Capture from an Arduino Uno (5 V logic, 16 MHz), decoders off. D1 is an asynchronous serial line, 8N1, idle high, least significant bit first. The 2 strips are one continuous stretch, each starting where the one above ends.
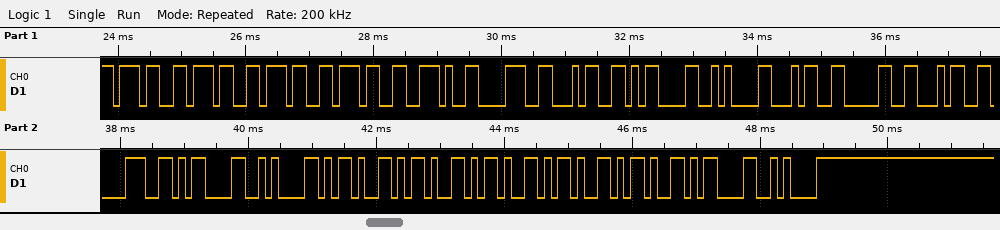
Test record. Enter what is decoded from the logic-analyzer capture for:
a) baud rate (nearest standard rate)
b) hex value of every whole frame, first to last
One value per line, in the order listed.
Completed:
9600 baud
37 37 37 37 2E 38 34 0D 0A 34 30 34 38 0D 0A 2D 2D 2D 2D 2D 0D 0A
